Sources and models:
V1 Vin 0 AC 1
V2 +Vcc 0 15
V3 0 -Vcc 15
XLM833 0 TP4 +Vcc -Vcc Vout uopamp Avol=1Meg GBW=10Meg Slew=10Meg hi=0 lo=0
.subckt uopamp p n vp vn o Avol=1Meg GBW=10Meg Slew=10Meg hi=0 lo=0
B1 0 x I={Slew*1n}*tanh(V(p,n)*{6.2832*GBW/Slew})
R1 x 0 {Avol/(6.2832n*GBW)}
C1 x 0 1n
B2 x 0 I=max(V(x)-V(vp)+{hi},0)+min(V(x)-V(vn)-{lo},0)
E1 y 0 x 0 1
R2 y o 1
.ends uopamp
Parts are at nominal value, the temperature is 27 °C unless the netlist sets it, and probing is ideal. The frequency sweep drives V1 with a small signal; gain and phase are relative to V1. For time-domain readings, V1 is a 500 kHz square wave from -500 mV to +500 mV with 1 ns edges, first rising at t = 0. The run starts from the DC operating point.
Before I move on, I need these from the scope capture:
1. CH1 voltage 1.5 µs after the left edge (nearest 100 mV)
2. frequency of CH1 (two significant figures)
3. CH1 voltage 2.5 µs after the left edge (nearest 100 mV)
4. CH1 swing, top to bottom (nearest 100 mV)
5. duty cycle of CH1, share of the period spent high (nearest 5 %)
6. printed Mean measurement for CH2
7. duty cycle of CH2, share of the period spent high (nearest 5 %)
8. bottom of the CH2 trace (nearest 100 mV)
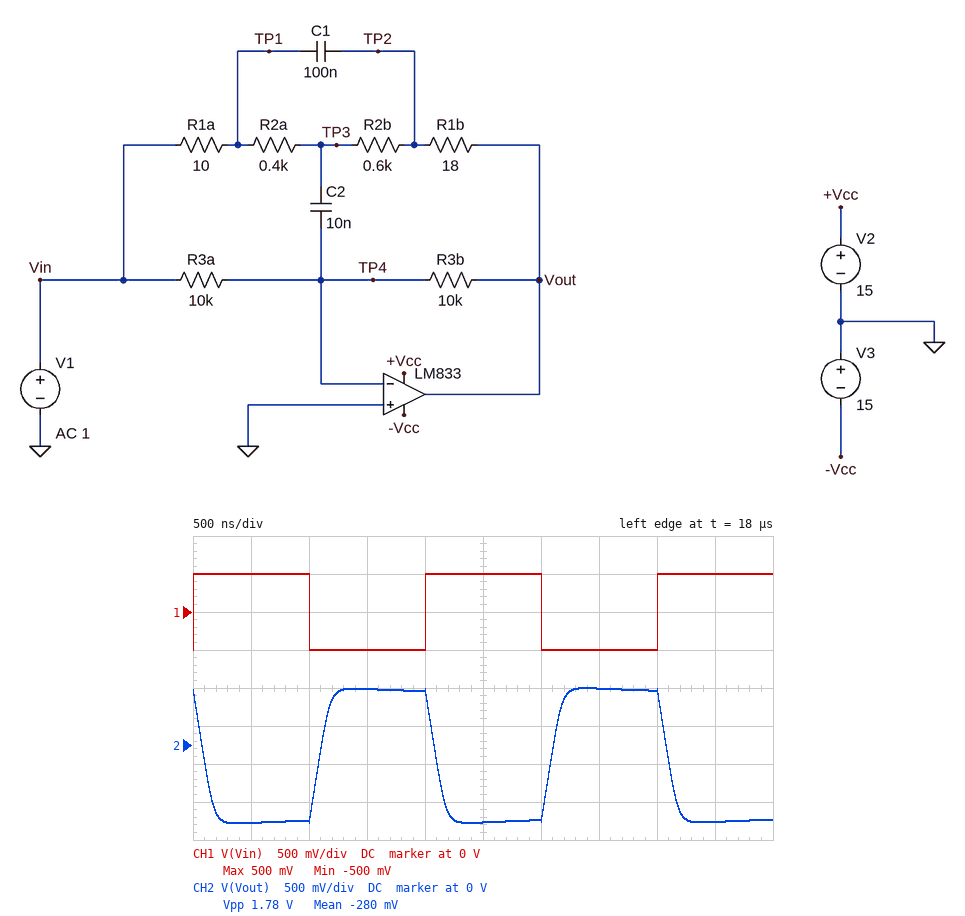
-500 mV
500 kHz
500 mV
1.0 V
50 %
-280 mV
50 %
-1.0 V
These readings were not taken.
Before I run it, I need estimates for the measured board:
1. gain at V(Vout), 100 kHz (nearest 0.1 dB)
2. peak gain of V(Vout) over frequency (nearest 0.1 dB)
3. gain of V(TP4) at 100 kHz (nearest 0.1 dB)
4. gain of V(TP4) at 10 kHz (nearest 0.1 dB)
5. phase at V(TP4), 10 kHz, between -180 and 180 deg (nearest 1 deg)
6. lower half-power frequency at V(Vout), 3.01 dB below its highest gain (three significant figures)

4.5 dB
4.8 dB
-35.2 dB
-56.9 dB
98 deg
3.32 kHz
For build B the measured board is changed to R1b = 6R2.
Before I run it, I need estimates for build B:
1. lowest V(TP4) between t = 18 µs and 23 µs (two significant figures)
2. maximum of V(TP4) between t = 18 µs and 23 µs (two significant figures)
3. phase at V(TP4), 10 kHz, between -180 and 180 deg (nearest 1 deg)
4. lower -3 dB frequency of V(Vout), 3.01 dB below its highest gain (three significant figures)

-420 mV
420 mV
92 deg
647 Hz
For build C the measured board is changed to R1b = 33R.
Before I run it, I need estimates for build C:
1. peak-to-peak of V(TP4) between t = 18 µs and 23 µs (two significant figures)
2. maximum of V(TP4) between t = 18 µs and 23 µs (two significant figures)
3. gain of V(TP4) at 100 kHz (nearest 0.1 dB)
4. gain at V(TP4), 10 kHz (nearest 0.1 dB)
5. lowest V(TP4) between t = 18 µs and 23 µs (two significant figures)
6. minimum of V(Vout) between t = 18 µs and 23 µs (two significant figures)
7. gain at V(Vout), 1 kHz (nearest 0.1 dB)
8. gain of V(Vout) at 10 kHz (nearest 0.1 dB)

1.5 V
760 mV
-31.1 dB
-56.8 dB
-760 mV
-1.7 V
0.3 dB
3.2 dB
